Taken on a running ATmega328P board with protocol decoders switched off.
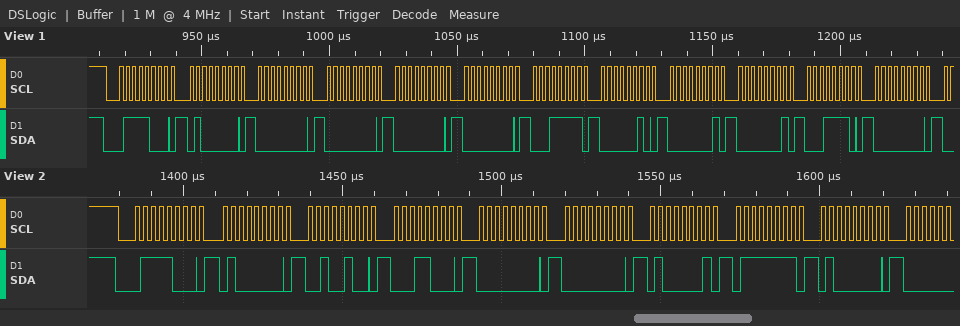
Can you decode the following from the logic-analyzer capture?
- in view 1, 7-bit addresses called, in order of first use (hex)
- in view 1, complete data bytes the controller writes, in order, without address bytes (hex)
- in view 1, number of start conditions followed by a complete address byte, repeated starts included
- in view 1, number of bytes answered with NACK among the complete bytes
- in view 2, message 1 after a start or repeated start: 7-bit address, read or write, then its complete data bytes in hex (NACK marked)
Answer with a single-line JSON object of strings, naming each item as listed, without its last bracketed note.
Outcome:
{"in view 1, 7-bit addresses called, in order of first use": "0x3C", "in view 1, complete data bytes the controller writes, in order, without address bytes": "40 00 00 00 00 1F 02 01 01 1E 00", "in view 1, number of start conditions followed by a complete address byte, repeated starts included": "1", "in view 1, number of bytes answered with NACK among the complete bytes": "0", "in view 2, message 1 after a start or repeated start: 7-bit address, read or write, then its complete data bytes in hex": "0x3C write: 40 24 18 00 00 41 7F 40"}
